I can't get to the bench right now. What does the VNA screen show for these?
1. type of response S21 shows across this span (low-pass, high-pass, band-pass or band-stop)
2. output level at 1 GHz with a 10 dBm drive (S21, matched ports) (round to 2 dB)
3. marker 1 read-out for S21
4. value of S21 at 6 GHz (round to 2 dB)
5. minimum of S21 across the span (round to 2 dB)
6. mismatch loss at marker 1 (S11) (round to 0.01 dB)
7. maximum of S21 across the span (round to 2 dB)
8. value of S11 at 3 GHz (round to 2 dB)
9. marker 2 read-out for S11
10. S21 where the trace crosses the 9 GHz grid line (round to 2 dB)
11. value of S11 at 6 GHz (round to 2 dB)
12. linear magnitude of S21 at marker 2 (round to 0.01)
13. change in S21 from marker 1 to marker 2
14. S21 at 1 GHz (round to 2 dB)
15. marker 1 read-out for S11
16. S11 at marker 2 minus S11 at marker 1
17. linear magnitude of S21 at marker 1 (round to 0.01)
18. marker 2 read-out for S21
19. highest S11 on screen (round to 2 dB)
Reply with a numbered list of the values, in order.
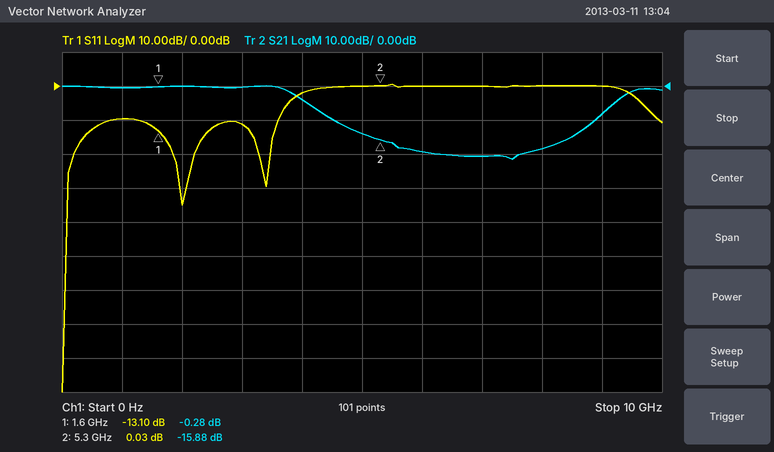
1. band-stop
2. 10 dBm
3. -0.28 dB
4. -20 dB
5. -22 dB
6. 0.22 dB
7. 0 dB
8. -12 dB
9. 0.03 dB
10. -8 dB
11. 0 dB
12. 0.16
13. -15.60 dB
14. 0 dB
15. -13.10 dB
16. 13.13 dB
17. 0.97
18. -15.88 dB
19. 0 dB
